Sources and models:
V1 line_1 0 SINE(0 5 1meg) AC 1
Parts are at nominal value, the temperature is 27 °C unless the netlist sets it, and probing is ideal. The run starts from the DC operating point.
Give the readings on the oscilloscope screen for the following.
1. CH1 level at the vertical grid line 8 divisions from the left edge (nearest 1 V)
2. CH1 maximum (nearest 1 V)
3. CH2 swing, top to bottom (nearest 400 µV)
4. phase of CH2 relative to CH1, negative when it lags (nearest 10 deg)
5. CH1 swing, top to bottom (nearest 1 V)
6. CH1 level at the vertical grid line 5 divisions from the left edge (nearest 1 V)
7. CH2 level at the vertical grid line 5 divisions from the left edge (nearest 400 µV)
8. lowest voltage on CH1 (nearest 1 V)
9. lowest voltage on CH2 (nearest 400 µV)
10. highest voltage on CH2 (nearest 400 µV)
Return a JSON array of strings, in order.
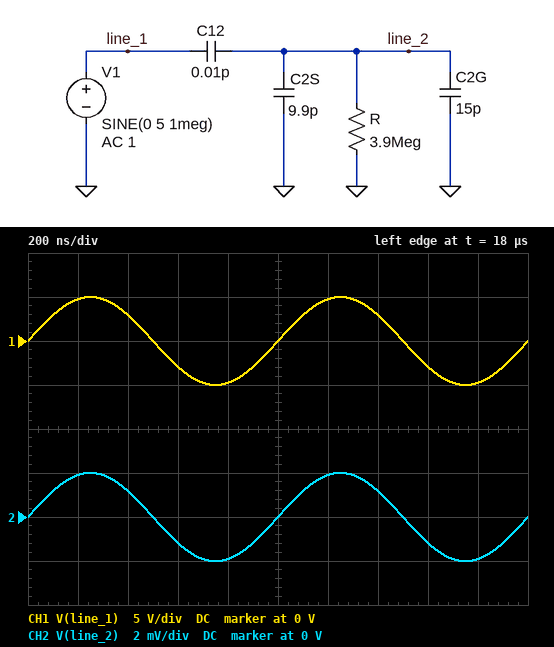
["-3 V", "5 V", "4.0 mV", "0 deg", "10 V", "0 V", "0 V", "-5 V", "-2.0 mV", "2.0 mV"]
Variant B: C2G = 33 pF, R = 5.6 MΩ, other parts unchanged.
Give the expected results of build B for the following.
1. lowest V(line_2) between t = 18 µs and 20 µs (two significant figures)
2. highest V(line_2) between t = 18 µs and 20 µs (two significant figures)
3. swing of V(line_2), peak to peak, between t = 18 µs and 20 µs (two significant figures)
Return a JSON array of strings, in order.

["-1.2 mV", "1.2 mV", "2.3 mV"]
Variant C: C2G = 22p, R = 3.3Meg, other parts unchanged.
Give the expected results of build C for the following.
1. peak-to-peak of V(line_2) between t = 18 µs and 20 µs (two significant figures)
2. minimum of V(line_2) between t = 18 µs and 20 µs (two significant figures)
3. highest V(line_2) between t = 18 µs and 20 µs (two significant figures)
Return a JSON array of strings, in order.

["3.1 mV", "-1.6 mV", "1.6 mV"]
